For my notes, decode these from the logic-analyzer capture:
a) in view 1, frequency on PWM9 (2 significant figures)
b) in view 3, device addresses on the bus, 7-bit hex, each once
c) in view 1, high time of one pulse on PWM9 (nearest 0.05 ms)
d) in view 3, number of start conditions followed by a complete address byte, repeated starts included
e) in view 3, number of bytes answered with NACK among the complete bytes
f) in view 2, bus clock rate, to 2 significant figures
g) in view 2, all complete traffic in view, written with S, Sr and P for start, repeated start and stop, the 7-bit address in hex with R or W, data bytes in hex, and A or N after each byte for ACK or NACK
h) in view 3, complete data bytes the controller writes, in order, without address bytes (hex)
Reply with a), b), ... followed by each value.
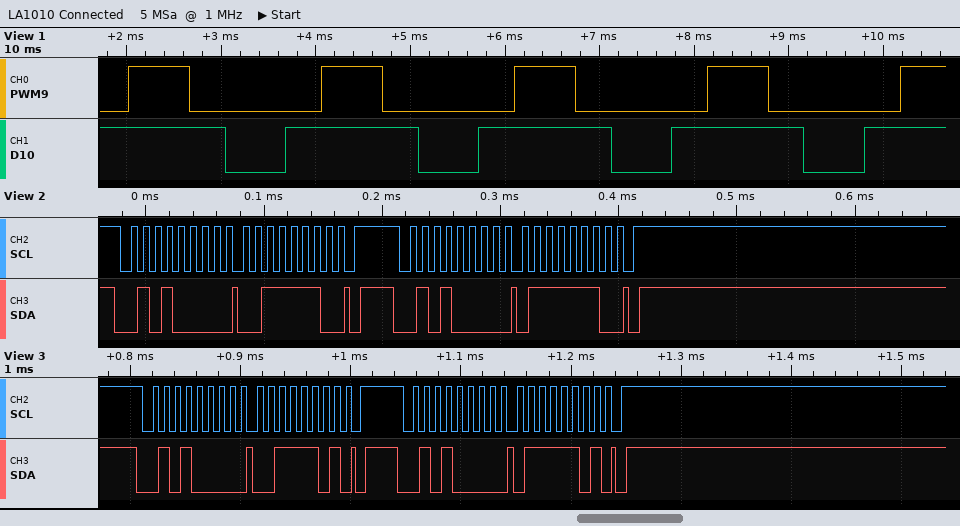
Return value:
a) 490 Hz
b) 0x28
c) 0.65 ms
d) 2
e) 0
f) 100 kHz
g) S 28W A 3E A P S 28W A 7E A P
h) 3D 7D
